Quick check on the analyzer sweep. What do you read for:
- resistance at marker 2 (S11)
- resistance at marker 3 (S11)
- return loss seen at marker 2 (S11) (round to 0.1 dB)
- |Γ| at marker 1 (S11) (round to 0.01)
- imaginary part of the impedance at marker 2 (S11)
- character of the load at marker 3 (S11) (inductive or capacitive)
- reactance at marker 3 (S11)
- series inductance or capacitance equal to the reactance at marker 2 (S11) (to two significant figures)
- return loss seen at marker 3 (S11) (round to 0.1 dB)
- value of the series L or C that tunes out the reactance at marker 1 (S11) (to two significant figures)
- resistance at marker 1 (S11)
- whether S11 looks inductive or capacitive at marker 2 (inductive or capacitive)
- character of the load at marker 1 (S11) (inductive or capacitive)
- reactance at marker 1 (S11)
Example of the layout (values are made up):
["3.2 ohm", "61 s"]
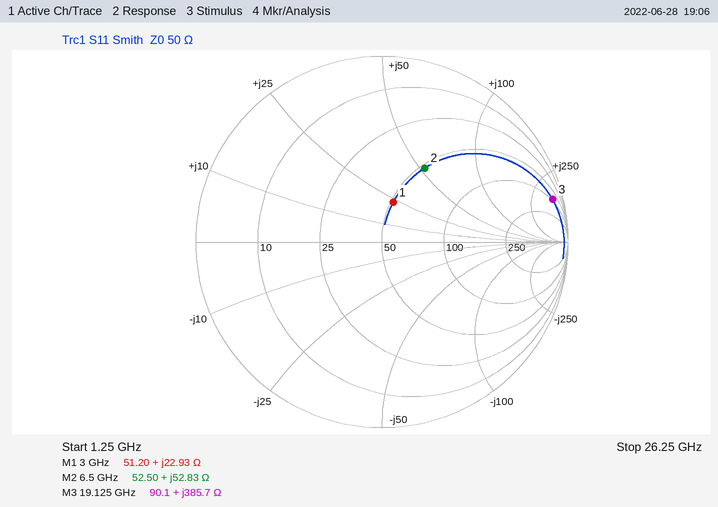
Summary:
["52.50 Ω", "90.1 Ω", "6.8 dB", "0.22", "+52.83 Ω", "inductive", "+385.7 Ω", "1.3 nH", "0.5 dB", "2.3 pF", "51.20 Ω", "inductive", "inductive", "+22.93 Ω"]
